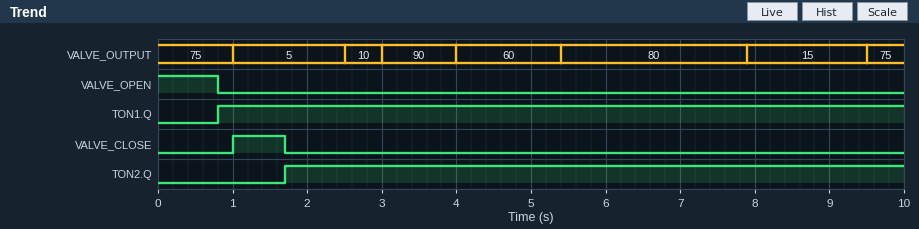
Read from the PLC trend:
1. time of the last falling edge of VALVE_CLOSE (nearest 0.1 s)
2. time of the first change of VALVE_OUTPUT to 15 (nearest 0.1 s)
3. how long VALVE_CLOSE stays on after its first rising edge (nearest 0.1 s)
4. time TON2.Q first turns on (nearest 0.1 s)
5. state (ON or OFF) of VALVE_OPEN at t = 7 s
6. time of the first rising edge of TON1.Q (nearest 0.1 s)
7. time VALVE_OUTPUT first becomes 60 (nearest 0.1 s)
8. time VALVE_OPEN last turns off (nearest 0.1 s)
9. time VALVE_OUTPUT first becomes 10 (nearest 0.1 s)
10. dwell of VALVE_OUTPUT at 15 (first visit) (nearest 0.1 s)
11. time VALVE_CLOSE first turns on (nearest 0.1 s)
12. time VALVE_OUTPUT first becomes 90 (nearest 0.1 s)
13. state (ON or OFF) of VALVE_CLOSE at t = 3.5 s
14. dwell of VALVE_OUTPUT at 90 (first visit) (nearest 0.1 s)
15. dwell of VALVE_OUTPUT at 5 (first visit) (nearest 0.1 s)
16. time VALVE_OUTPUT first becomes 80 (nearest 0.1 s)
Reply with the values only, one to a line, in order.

1.7 s
7.9 s
0.7 s
1.7 s
OFF
0.8 s
4.0 s
0.8 s
2.5 s
1.6 s
1.0 s
3.0 s
OFF
1.0 s
1.5 s
5.4 s
